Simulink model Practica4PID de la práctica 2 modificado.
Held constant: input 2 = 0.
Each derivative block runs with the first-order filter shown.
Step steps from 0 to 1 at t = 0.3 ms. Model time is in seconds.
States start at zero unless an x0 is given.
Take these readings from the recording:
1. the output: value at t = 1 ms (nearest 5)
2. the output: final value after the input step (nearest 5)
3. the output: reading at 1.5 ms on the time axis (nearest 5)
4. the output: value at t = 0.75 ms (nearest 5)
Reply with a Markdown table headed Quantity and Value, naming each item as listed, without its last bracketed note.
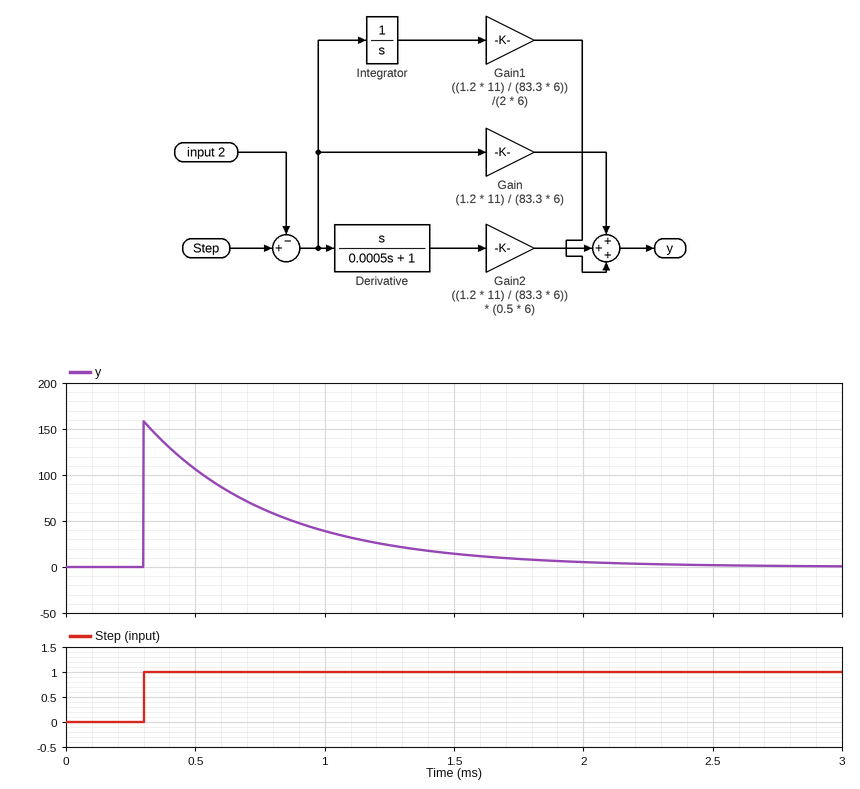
| Quantity | Value |
|---|---|
| the output: value at t = 1 ms | 40 |
| the output: final value after the input step | 0 |
| the output: reading at 1.5 ms on the time axis | 15 |
| the output: value at t = 0.75 ms | 65 |
